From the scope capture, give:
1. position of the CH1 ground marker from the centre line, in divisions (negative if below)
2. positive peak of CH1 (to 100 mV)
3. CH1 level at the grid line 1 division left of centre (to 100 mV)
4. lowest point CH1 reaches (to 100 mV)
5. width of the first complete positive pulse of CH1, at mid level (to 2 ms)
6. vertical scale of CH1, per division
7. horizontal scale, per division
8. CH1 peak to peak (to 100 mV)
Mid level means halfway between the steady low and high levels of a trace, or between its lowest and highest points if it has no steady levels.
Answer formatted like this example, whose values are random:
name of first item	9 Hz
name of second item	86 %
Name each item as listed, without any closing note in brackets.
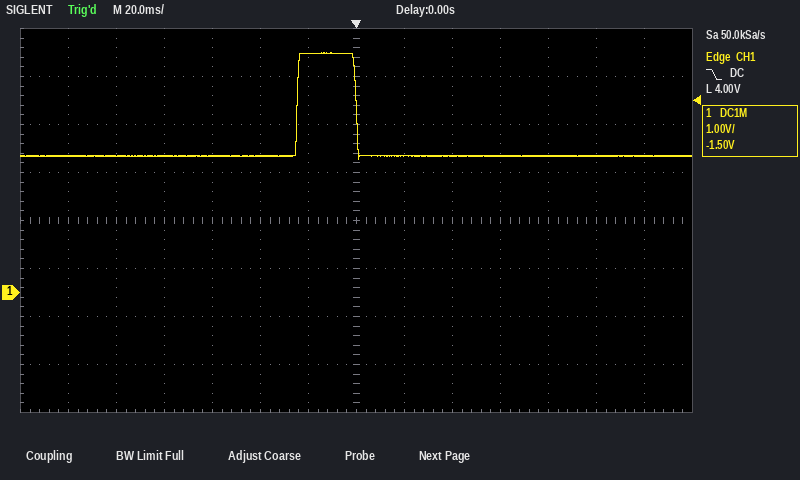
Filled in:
position of the CH1 ground marker from the centre line, in divisions	-1.5 div
positive peak of CH1	5.0 V
CH1 level at the grid line 1 division left of centre	5.0 V
lowest point CH1 reaches	2.8 V
width of the first complete positive pulse of CH1, at mid level	24 ms
vertical scale of CH1, per division	1 V
horizontal scale, per division	20 ms
CH1 peak to peak	2.2 V
